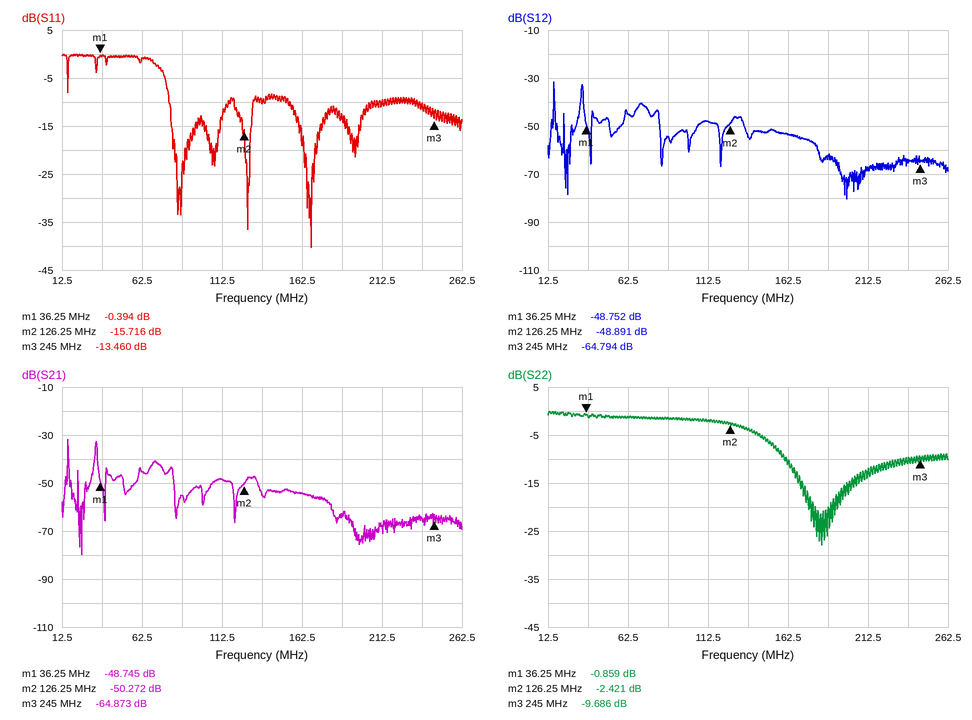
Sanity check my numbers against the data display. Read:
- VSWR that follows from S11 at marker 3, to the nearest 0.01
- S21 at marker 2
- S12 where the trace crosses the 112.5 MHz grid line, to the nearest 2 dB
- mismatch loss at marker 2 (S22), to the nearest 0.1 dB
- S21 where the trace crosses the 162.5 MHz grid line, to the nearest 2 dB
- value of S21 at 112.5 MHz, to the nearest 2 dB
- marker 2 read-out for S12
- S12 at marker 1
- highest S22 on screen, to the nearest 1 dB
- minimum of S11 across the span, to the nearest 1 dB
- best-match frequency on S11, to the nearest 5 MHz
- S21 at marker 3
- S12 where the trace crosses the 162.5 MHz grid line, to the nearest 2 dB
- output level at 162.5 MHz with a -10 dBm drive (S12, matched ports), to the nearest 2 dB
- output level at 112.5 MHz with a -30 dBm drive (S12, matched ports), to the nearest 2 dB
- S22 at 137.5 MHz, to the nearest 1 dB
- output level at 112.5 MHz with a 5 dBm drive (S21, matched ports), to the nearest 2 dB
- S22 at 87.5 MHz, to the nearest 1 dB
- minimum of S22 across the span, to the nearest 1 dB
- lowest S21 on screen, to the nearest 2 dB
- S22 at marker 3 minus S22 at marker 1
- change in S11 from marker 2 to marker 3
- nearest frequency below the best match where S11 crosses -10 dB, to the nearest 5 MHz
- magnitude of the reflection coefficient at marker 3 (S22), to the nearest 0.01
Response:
1.54
-50.272 dB
-48 dB
3.7 dB
-54 dB
-48 dB
-48.891 dB
-48.752 dB
0 dB
-40 dB
170 MHz
-64.873 dB
-54 dB
-64 dBm
-78 dBm
-4 dB
-44 dBm
-1 dB
-28 dB
-80 dB
-8.827 dB
2.256 dB
155 MHz
0.33
